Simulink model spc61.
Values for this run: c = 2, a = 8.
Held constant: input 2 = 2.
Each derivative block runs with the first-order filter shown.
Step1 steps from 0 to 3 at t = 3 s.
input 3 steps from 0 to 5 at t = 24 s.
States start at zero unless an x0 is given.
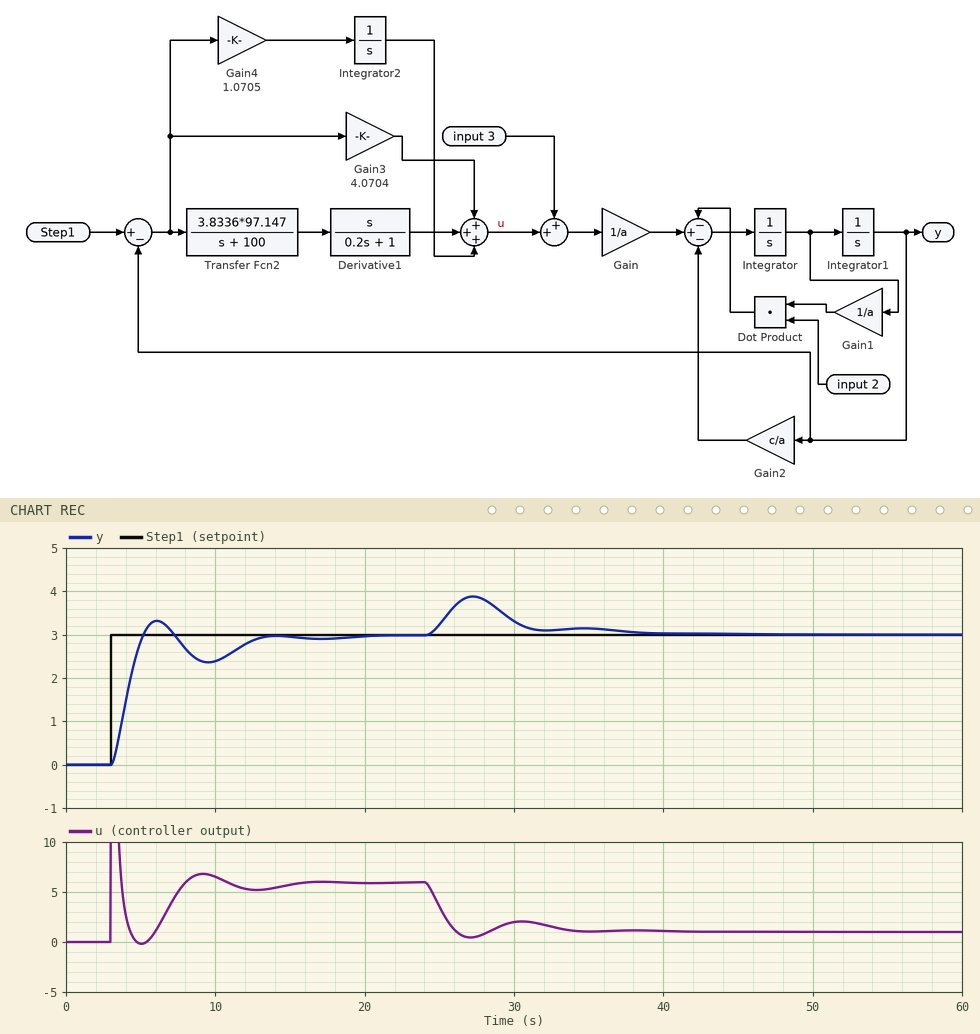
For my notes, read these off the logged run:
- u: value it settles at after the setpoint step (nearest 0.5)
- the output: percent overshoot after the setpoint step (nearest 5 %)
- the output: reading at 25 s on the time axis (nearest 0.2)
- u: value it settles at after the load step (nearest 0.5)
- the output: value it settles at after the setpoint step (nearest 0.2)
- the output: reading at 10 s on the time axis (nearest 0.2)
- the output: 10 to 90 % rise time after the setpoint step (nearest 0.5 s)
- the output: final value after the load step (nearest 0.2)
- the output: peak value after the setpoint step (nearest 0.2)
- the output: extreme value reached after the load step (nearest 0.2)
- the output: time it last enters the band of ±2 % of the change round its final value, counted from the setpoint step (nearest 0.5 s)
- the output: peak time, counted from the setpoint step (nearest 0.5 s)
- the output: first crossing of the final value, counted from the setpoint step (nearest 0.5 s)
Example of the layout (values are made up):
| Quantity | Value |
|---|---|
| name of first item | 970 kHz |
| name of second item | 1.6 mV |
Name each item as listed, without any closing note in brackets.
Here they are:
| Quantity | Value |
|---|---|
| u: value it settles at after the setpoint step | 6.0 |
| the output: percent overshoot after the setpoint step | 10 % |
| the output: reading at 25 s on the time axis | 3.2 |
| u: value it settles at after the load step | 1.0 |
| the output: value it settles at after the setpoint step | 3.0 |
| the output: reading at 10 s on the time axis | 2.4 |
| the output: 10 to 90 % rise time after the setpoint step | 1.5 s |
| the output: final value after the load step | 3.0 |
| the output: peak value after the setpoint step | 3.4 |
| the output: extreme value reached after the load step | 3.8 |
| the output: time it last enters the band of ±2 % of the change round its final value, counted from the setpoint step | 16.0 s |
| the output: peak time, counted from the setpoint step | 3.0 s |
| the output: first crossing of the final value, counted from the setpoint step | 2.0 s |
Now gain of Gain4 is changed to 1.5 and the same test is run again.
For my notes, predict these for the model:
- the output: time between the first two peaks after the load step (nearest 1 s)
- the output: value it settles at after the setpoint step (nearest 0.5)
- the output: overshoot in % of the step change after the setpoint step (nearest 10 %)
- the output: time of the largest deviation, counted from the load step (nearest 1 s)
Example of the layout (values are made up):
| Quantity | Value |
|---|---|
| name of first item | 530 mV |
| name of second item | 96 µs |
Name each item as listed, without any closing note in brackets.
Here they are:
| Quantity | Value |
|---|---|
| the output: time between the first two peaks after the load step | 8 s |
| the output: value it settles at after the setpoint step | 3.0 |
| the output: overshoot in % of the step change after the setpoint step | 20 % |
| the output: time of the largest deviation, counted from the load step | 3 s |
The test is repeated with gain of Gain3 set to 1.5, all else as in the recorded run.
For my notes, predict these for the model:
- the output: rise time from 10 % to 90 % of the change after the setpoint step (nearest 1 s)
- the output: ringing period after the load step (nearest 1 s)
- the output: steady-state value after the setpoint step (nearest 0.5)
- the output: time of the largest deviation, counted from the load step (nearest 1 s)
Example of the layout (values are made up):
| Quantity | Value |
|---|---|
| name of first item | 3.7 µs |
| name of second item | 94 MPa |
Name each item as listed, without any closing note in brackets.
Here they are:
| Quantity | Value |
|---|---|
| the output: rise time from 10 % to 90 % of the change after the setpoint step | 3 s |
| the output: ringing period after the load step | 12 s |
| the output: steady-state value after the setpoint step | 3.0 |
| the output: time of the largest deviation, counted from the load step | 4 s |
